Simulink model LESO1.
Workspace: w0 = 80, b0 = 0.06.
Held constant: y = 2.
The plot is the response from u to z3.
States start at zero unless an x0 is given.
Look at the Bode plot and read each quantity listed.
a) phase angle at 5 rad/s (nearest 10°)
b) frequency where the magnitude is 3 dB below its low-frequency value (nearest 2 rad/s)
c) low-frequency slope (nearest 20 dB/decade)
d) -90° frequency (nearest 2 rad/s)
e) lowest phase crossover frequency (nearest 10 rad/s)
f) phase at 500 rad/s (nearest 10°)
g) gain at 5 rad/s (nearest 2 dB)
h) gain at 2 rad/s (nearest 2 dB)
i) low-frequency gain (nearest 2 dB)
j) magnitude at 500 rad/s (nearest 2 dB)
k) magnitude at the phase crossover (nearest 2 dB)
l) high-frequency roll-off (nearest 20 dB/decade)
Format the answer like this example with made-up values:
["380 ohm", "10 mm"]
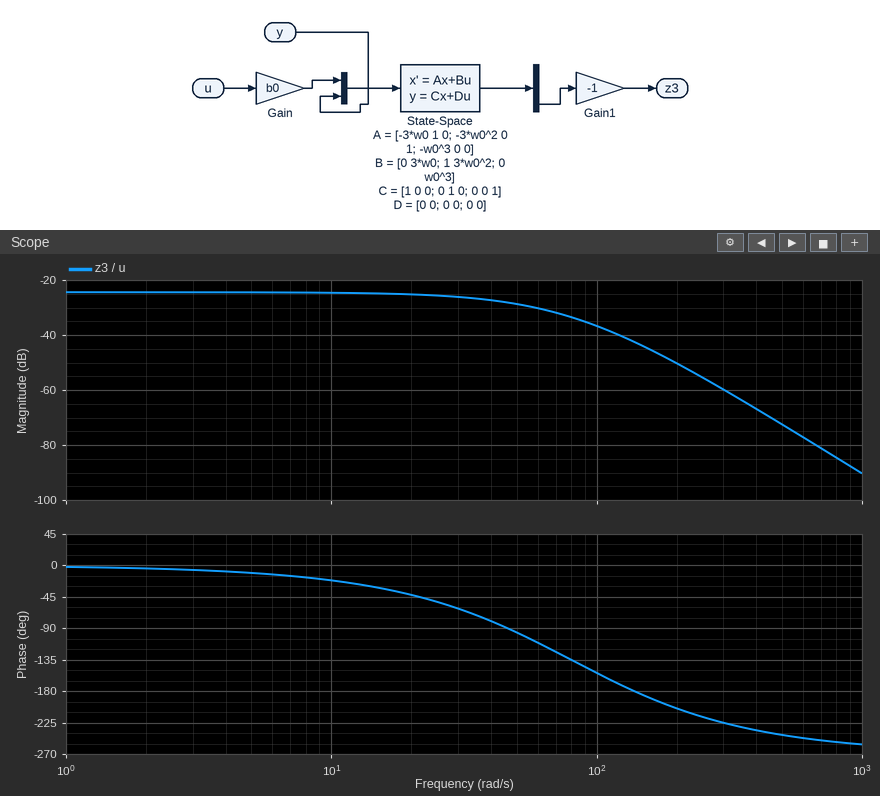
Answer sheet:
["-10°", "40 rad/s", "0 dB/decade", "46 rad/s", "140 rad/s", "-240°", "-24 dB", "-24 dB", "-24 dB", "-72 dB", "-42 dB", "-60 dB/decade"]
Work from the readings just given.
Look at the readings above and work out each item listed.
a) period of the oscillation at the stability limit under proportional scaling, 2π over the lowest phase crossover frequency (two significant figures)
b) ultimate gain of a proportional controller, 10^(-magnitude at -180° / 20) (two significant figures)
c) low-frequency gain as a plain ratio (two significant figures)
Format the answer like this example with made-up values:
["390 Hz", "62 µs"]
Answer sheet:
["0.045 s", "130", "0.063"]
